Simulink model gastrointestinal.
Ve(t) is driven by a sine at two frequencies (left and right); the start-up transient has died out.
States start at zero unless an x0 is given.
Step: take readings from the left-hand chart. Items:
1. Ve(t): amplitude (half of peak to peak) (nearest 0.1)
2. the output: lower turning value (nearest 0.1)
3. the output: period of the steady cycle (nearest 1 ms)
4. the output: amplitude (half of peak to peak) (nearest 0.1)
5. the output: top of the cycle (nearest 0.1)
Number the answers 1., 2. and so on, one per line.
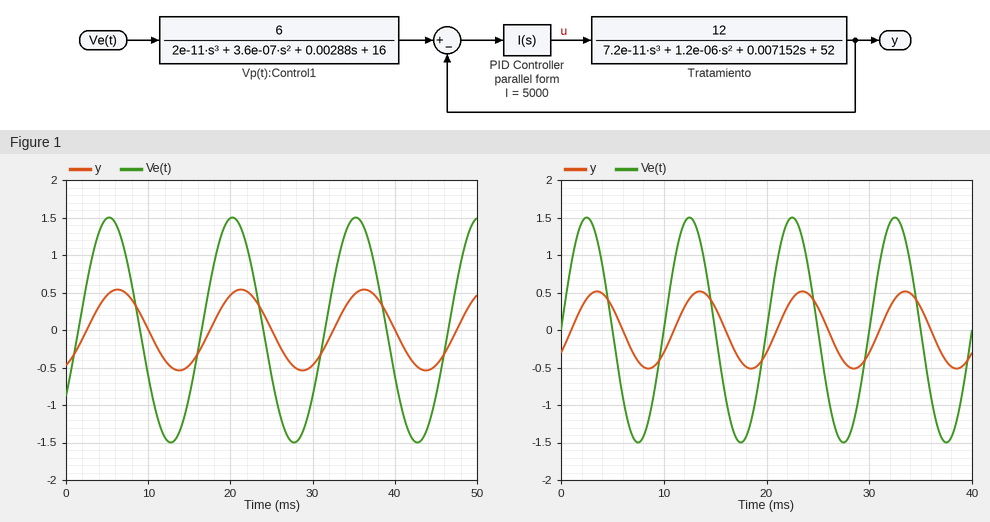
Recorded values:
1. 1.5
2. -0.5
3. 15 ms
4. 0.5
5. 0.5
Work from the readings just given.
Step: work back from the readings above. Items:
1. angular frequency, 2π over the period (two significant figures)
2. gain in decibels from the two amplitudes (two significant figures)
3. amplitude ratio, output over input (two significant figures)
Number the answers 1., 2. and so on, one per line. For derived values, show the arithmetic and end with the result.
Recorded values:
1. 2π / 15 = 0.42 rad/ms
2. 20 log10(0.5 / 1.5) = -9.5 dB
3. 0.5 / 1.5 = 0.33
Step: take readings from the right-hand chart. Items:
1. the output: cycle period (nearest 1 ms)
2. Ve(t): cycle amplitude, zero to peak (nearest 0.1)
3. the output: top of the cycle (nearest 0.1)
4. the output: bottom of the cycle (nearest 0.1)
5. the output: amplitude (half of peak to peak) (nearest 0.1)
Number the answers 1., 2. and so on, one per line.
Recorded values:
1. 10 ms
2. 1.5
3. 0.5
4. -0.5
5. 0.5
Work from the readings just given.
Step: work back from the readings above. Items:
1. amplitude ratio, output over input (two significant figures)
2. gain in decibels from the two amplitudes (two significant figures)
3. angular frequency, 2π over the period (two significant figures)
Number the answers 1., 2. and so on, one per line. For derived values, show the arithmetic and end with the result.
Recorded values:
1. 0.5 / 1.5 = 0.33
2. 20 log10(0.5 / 1.5) = -9.5 dB
3. 2π / 10 = 0.63 rad/ms
